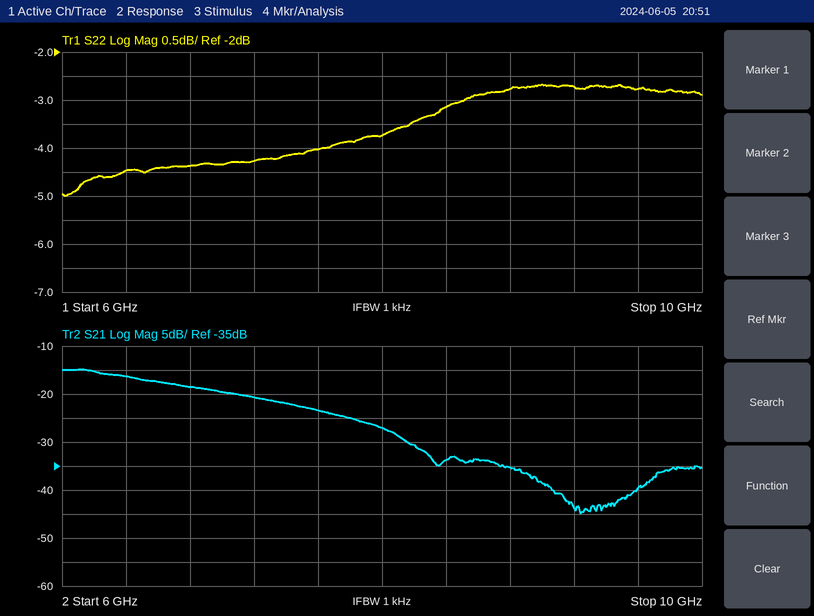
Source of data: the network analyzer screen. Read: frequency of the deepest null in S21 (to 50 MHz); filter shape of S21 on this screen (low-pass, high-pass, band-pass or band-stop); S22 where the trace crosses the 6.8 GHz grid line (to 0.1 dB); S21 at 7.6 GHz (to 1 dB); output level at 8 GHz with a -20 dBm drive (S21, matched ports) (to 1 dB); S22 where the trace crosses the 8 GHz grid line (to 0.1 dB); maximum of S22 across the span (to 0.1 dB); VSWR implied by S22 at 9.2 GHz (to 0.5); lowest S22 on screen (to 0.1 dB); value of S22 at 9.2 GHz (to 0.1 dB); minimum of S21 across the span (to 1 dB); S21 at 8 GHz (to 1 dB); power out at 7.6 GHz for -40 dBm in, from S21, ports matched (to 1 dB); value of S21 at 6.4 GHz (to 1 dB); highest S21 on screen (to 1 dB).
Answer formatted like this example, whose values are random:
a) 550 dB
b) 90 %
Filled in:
a) 9.25 GHz
b) low-pass
c) -4.4 dB
d) -23 dB
e) -47 dBm
f) -3.7 dB
g) -2.7 dB
h) 6.5
i) -5.0 dB
j) -2.7 dB
k) -45 dB
l) -27 dB
m) -63 dBm
n) -16 dB
o) -15 dB
